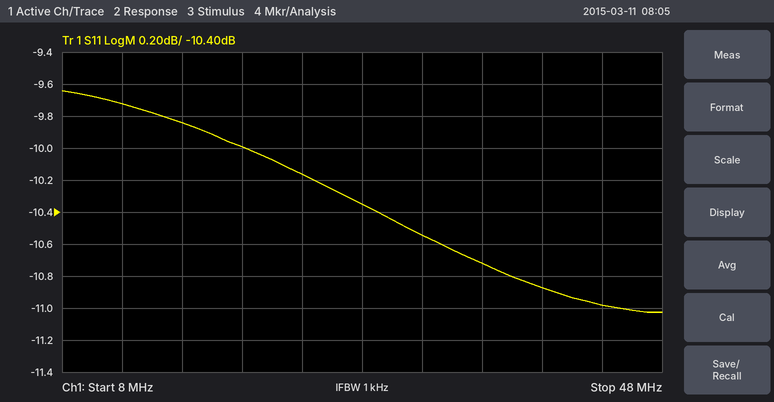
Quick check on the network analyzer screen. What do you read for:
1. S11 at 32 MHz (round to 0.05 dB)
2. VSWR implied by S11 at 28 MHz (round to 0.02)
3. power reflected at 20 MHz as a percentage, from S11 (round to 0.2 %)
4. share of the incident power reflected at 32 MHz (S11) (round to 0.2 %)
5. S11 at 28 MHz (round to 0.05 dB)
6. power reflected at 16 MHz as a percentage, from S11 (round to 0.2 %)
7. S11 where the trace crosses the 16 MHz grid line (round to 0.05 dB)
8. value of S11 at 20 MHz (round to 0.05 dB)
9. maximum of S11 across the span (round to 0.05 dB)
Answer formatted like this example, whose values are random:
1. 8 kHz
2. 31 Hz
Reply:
1. -10.55 dB
2. 1.88
3. 10.0 %
4. 8.8 %
5. -10.35 dB
6. 10.4 %
7. -9.85 dB
8. -10.00 dB
9. -9.65 dB
